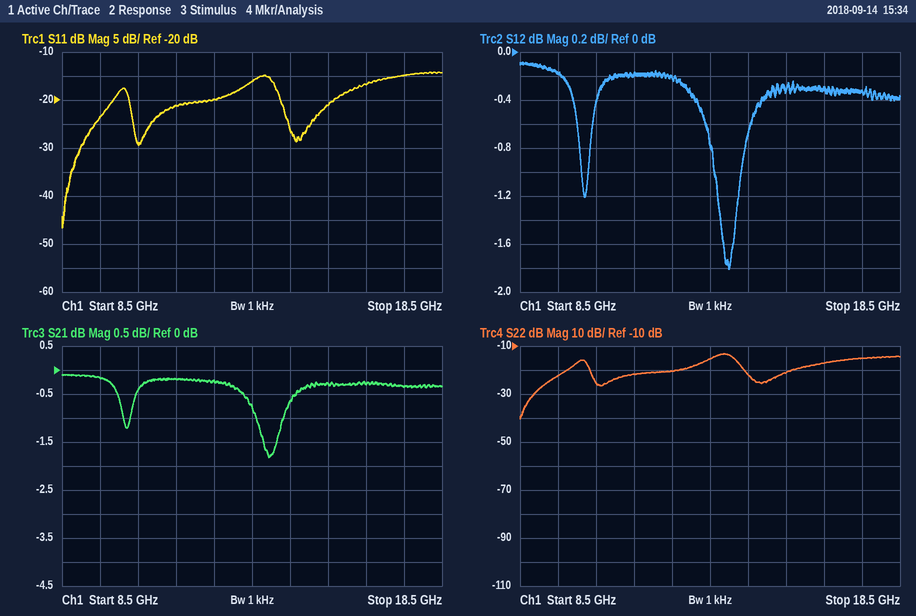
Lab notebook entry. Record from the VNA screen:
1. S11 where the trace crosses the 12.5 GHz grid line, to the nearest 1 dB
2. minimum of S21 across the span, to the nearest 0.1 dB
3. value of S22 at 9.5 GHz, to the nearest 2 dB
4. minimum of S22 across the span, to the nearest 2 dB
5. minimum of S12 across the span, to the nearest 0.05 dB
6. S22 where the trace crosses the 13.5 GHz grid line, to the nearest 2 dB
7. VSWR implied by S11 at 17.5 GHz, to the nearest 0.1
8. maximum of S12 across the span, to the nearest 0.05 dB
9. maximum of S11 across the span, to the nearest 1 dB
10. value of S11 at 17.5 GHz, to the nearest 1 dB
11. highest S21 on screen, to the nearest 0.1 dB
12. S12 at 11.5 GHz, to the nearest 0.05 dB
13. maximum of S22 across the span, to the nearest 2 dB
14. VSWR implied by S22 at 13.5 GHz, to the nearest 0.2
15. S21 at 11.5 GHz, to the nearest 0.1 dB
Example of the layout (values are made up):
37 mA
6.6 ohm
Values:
-20 dB
-1.8 dB
-22 dB
-40 dB
-1.80 dB
-16 dB
1.4
-0.10 dB
-14 dB
-15 dB
-0.1 dB
-0.20 dB
-14 dB
1.4
-0.2 dB
